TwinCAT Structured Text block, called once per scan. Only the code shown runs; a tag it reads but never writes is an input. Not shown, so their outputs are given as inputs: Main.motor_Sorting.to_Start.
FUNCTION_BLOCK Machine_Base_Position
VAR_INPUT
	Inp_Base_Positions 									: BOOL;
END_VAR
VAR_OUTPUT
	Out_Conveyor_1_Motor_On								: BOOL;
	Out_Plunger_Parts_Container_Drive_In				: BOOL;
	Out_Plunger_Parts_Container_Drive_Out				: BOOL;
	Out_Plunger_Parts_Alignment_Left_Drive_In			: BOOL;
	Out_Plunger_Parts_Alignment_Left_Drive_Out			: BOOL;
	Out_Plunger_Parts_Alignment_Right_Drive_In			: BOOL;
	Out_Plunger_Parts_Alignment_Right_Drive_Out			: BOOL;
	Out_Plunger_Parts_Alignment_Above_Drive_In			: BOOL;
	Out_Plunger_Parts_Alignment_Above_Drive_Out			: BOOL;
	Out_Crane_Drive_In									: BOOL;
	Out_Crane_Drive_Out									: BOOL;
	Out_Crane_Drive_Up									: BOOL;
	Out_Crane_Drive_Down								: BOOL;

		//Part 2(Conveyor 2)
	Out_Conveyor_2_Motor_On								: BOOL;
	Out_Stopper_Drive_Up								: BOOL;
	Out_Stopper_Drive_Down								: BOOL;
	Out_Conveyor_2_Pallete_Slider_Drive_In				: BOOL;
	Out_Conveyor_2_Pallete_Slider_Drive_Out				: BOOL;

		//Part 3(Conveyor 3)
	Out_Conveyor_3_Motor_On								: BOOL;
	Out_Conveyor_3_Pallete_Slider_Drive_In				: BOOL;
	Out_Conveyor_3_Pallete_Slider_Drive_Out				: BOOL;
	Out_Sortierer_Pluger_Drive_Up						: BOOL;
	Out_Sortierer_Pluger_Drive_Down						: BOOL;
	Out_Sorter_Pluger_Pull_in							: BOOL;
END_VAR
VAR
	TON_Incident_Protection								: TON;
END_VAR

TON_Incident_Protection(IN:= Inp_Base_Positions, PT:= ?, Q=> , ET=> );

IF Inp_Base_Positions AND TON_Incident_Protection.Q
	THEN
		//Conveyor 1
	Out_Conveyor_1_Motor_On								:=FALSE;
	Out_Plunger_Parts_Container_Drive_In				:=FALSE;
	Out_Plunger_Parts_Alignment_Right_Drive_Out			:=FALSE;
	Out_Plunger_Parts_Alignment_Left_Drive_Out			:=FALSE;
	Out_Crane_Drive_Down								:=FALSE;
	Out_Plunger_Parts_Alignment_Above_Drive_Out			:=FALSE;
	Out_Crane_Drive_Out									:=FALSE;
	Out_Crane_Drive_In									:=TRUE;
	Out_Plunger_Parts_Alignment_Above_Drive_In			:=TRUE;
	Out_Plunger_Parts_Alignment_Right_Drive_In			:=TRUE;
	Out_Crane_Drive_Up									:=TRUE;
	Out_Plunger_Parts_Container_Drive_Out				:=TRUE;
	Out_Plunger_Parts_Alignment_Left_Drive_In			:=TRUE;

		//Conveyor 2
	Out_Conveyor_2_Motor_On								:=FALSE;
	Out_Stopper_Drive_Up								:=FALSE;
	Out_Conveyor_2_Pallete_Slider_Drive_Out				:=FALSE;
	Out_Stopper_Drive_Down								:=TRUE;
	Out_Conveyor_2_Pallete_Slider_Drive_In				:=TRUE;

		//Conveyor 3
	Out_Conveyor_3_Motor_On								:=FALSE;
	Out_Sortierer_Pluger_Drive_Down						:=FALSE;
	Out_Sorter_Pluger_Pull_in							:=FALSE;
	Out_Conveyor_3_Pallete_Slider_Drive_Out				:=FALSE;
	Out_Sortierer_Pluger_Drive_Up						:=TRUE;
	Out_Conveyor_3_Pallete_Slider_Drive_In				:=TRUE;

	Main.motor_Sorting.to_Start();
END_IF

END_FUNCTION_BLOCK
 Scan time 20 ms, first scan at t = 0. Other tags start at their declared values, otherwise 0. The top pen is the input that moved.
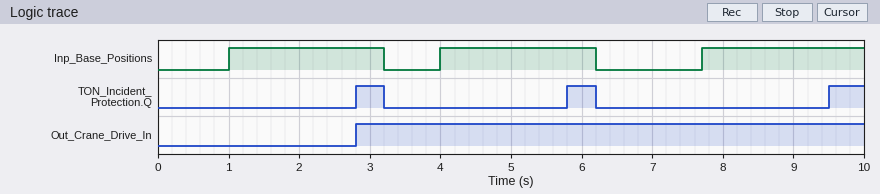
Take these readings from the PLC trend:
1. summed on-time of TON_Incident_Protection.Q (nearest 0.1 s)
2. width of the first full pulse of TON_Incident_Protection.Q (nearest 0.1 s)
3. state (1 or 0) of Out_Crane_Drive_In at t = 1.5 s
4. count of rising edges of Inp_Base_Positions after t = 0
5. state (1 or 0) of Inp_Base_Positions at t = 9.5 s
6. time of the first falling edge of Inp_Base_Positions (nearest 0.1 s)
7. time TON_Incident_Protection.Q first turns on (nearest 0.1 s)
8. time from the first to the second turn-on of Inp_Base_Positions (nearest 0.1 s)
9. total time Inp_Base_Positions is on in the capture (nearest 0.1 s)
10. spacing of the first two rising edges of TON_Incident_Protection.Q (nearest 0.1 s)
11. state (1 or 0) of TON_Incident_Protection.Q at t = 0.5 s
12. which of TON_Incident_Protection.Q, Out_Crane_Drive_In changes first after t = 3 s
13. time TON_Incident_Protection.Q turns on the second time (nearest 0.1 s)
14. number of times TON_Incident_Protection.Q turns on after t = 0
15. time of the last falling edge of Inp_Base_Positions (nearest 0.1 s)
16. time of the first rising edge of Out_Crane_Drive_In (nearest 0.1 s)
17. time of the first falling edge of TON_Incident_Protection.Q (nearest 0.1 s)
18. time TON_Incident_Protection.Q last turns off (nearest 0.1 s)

1.3 s
0.4 s
0
3
1
3.2 s
2.8 s
3.0 s
6.7 s
3.0 s
0
TON_Incident_Protection.Q
5.8 s
3
6.2 s
2.8 s
3.2 s
6.2 s
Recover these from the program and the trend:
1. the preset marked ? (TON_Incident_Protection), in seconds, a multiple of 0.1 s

1.8 s
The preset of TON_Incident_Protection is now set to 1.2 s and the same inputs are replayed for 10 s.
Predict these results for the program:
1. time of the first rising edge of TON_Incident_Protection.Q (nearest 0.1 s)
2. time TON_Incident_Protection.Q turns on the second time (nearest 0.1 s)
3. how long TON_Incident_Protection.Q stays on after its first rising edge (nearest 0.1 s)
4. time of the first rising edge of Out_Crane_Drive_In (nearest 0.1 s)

2.2 s
5.2 s
1.0 s
2.2 s
